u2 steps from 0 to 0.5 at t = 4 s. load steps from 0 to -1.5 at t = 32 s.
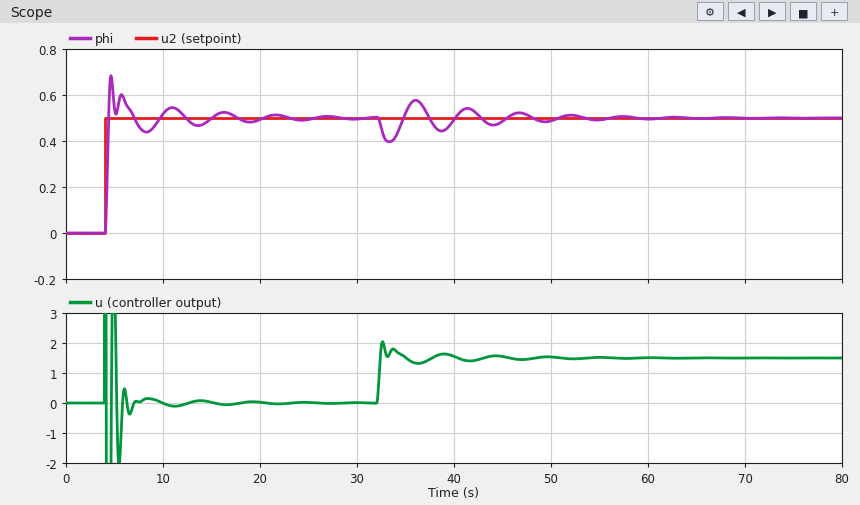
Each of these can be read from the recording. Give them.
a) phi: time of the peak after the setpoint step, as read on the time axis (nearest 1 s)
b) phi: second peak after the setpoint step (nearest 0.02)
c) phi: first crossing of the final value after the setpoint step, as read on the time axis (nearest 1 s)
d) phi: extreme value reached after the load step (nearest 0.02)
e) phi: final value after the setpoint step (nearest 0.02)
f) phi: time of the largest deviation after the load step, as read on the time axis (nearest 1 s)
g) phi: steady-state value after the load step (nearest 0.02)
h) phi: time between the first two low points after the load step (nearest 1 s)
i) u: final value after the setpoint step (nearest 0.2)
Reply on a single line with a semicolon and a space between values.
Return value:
5 s; 0.60; 4 s; 0.40; 0.50; 33 s; 0.50; 5 s; 0.0
